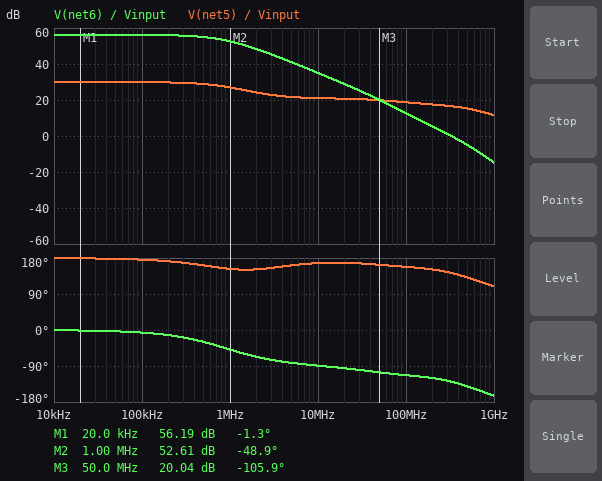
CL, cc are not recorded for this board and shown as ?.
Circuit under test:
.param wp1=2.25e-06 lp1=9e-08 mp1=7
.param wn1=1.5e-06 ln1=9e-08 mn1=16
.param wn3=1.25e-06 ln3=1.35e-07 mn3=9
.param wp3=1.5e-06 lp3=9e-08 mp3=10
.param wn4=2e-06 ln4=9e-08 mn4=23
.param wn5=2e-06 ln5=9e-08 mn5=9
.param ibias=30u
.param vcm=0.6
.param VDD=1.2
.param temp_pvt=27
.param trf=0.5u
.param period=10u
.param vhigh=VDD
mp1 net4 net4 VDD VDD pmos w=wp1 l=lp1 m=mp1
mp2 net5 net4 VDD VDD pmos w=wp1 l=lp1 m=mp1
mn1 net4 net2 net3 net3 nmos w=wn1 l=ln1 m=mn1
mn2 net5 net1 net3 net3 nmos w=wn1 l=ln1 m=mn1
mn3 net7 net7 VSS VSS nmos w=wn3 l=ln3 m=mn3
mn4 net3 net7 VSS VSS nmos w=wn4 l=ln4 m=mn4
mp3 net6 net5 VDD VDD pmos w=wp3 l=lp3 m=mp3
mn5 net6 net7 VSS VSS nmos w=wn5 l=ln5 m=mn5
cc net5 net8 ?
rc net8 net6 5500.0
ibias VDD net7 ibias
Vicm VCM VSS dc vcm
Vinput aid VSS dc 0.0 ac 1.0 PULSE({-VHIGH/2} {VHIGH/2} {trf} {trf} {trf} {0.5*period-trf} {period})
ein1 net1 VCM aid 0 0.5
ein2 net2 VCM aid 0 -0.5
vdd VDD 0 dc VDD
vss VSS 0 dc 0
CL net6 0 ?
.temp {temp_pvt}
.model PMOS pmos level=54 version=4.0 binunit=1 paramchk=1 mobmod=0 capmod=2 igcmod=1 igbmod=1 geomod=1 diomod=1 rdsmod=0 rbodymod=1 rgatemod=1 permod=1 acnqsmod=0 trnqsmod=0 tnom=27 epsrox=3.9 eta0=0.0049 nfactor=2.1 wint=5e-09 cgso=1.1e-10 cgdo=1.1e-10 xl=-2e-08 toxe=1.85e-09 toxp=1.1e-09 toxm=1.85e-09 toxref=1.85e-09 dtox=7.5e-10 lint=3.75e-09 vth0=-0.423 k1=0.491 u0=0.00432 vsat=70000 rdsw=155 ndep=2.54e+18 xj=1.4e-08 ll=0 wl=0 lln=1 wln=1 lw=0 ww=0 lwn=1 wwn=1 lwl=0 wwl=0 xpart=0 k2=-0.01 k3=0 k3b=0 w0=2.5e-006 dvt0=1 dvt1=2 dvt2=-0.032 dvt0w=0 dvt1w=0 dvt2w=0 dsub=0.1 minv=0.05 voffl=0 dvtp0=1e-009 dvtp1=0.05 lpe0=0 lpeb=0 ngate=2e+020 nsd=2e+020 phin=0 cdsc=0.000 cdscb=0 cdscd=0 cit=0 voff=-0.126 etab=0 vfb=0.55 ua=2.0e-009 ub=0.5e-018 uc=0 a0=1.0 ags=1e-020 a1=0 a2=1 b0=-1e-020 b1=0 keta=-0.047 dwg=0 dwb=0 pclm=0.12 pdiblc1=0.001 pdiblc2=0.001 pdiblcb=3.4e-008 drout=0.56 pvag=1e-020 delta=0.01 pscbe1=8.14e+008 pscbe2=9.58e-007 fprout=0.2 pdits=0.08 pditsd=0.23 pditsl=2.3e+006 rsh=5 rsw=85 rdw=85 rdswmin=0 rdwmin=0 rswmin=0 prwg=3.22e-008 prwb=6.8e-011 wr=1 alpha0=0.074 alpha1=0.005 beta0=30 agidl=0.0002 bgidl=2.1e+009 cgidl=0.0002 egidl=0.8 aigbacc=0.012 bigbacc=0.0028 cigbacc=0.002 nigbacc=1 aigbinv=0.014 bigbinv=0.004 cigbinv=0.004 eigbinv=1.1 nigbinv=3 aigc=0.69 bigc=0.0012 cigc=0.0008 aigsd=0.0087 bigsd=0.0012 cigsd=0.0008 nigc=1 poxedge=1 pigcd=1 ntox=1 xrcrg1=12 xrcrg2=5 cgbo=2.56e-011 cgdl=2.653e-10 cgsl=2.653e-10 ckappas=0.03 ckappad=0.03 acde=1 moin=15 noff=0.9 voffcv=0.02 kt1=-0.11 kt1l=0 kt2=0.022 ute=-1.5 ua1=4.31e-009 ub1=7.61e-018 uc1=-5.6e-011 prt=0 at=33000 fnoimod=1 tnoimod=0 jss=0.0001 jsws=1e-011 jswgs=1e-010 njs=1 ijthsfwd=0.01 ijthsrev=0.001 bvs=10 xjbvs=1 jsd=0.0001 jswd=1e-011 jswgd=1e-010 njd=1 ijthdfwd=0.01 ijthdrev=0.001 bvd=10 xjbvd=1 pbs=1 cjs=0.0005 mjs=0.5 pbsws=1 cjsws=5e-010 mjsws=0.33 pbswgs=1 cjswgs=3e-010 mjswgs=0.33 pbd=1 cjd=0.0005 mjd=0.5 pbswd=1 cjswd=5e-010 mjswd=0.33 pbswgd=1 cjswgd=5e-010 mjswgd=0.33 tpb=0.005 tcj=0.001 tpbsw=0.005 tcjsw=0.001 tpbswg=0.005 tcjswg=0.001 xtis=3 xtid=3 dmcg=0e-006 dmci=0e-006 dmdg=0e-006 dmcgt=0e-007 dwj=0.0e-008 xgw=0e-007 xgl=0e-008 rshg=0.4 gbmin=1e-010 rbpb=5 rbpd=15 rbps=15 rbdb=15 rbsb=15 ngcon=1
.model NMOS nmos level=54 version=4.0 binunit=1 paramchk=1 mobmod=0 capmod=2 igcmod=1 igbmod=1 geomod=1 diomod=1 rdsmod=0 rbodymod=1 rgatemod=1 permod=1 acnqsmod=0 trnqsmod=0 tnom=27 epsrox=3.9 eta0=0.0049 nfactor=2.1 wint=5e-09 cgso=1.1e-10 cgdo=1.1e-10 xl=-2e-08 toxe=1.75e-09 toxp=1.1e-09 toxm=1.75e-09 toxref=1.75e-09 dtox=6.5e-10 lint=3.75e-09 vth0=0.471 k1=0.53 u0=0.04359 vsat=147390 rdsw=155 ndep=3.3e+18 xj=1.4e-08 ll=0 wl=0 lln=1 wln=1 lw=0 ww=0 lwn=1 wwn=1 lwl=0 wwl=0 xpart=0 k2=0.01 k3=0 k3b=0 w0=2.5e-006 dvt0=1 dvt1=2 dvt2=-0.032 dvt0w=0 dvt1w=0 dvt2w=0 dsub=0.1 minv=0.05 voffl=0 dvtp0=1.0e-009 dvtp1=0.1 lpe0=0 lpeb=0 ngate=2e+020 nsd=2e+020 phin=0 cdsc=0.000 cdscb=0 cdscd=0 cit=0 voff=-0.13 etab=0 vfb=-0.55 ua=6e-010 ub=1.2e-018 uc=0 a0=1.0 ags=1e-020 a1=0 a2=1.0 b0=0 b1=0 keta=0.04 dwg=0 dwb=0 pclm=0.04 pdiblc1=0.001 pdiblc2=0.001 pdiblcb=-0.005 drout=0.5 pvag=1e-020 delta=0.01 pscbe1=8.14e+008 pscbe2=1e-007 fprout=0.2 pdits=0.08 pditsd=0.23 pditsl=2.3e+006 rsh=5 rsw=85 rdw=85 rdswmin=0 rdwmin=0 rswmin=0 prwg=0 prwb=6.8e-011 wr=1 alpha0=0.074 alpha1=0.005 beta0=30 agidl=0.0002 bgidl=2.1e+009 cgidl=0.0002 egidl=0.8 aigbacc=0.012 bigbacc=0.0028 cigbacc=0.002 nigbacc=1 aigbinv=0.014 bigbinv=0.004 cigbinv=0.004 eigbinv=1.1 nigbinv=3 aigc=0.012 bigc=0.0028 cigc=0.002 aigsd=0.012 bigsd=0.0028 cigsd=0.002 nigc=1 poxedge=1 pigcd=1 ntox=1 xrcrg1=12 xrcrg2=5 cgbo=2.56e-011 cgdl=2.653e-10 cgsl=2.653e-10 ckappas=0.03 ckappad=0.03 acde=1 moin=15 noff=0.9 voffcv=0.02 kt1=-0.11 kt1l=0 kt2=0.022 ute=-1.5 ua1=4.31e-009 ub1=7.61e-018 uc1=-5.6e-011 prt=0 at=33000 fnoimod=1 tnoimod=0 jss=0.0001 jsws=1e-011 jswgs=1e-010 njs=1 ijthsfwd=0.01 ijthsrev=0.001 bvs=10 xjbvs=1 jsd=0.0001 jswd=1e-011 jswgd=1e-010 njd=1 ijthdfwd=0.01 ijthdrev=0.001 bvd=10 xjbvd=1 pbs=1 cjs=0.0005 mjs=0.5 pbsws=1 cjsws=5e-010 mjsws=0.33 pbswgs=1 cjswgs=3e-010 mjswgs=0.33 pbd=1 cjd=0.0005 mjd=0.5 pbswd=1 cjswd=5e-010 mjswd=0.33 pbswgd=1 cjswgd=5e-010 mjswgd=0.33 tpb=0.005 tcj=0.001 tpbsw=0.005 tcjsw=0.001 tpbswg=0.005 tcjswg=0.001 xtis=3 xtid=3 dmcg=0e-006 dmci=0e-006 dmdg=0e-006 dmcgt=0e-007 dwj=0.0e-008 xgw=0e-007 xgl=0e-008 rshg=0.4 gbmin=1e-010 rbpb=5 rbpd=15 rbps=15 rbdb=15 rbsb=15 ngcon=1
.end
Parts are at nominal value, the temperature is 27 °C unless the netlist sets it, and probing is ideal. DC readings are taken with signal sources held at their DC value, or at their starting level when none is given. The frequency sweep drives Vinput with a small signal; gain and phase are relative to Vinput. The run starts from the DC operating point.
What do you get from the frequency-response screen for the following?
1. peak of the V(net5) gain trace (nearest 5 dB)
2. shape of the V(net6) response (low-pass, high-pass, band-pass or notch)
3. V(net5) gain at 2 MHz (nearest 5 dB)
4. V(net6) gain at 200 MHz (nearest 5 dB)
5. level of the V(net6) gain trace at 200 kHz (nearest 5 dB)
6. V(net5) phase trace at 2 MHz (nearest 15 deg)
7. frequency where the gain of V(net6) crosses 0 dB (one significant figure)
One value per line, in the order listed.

30 dB
low-pass
25 dB
5 dB
55 dB
150 deg
300 MHz
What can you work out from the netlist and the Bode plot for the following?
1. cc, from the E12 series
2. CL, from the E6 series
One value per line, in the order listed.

330 fF
3.3 pF
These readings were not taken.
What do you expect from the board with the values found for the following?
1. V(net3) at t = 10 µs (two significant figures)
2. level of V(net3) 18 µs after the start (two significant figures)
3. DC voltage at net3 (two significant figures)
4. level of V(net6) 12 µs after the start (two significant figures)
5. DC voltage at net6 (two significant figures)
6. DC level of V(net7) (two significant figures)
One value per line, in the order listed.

450 mV
450 mV
200 mV
1.2 V
730 mV
410 mV
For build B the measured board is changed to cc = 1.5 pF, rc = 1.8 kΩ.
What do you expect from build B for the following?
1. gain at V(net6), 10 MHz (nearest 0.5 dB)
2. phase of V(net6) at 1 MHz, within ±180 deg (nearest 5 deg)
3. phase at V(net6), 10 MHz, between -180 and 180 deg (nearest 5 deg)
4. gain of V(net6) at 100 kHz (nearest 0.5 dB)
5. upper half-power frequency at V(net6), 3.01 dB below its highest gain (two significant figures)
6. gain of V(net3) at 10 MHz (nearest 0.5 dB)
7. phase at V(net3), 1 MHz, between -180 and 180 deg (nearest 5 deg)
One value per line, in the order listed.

24.5 dB
-75 deg
-95 deg
55.5 dB
260 kHz
-28.0 dB
135 deg
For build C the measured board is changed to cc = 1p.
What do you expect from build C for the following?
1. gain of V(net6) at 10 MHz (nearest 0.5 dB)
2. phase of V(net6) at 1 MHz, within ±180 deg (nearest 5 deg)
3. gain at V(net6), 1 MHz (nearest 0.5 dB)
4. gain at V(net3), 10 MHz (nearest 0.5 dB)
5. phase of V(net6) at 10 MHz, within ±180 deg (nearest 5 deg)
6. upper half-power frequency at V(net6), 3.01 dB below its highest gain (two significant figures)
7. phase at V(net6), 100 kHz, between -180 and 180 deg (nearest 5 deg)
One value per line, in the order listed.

28.0 dB
-70 deg
47.0 dB
-25.0 dB
-85 deg
370 kHz
-15 deg
